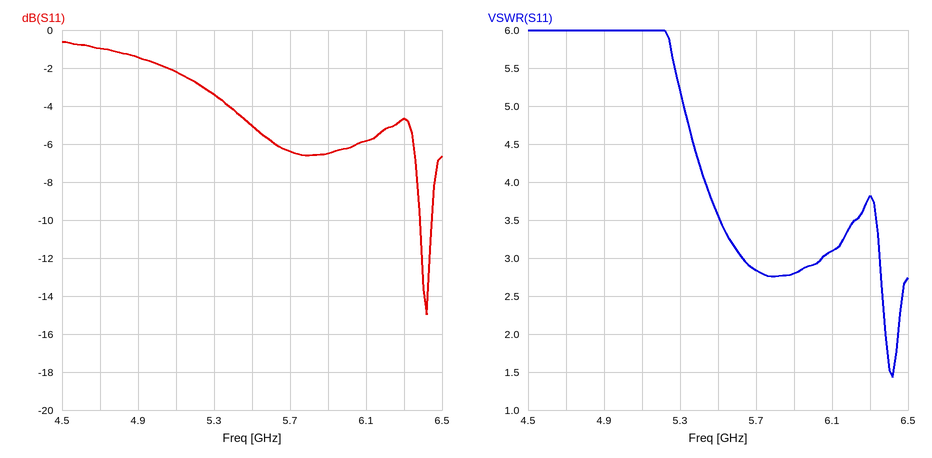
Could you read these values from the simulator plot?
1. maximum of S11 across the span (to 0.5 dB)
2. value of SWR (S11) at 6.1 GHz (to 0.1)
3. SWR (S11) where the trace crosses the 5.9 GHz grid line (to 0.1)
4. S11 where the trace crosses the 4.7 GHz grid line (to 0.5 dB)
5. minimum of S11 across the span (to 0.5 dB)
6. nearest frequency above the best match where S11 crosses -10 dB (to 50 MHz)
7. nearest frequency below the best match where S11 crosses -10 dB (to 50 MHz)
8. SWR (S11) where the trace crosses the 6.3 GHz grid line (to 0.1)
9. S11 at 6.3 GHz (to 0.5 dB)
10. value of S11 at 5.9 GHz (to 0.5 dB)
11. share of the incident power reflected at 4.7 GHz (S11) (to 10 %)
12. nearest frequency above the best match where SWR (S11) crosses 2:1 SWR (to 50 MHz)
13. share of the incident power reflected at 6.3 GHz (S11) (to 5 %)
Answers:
-0.5 dB
3.1
2.8
-1.0 dB
-15.0 dB
6.45 GHz
6.40 GHz
3.8
-4.5 dB
-6.5 dB
80 %
6.45 GHz
35 %
